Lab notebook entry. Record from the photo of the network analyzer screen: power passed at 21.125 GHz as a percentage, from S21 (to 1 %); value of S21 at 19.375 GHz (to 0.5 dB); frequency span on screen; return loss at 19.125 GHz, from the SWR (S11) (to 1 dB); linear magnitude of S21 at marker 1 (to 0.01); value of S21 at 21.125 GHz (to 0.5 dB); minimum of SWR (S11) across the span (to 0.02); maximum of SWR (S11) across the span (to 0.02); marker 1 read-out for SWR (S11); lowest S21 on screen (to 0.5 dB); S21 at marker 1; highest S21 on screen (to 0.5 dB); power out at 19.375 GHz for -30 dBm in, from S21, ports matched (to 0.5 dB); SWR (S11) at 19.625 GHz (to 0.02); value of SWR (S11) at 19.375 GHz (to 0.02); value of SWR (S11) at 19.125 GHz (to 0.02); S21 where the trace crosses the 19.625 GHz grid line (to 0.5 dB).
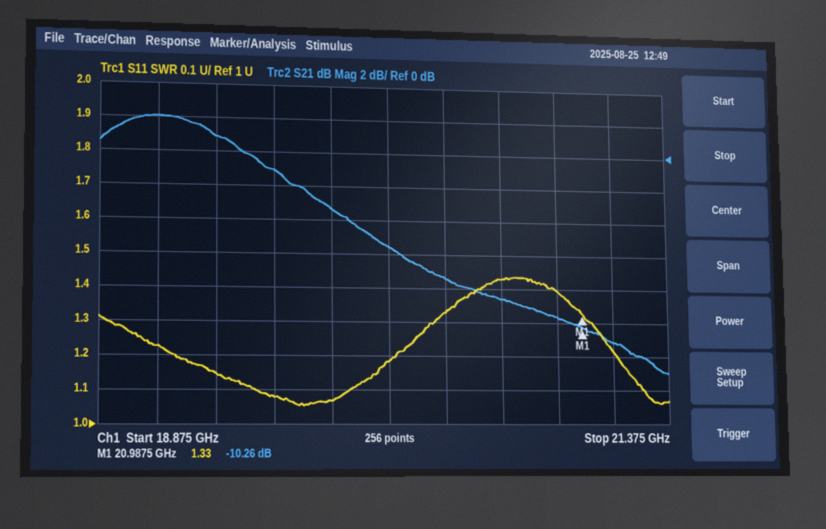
8 %
1.0 dB
2.5 GHz
20 dB
0.31
-11.0 dB
1.06
1.44
1.33
-13.0 dB
-10.26 dB
2.0 dB
-29.0 dBm
1.08
1.14
1.22
-1.0 dB
